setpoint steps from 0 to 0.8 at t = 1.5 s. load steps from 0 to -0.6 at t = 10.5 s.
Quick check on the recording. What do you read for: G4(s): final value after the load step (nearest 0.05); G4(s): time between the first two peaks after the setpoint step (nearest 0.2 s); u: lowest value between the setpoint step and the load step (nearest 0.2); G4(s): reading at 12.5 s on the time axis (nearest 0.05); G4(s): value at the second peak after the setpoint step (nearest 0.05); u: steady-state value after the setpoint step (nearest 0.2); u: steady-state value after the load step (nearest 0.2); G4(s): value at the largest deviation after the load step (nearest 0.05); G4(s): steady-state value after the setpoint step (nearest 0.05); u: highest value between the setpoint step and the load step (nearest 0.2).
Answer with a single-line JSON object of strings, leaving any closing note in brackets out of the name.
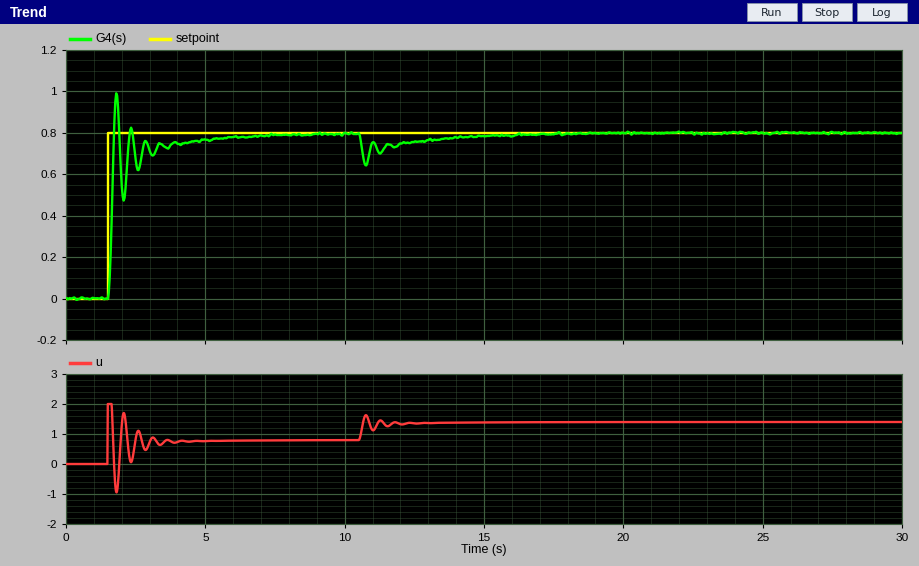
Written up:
{"G4(s): final value after the load step": "0.80", "G4(s): time between the first two peaks after the setpoint step": "0.6 s", "u: lowest value between the setpoint step and the load step": "-1.0", "G4(s): reading at 12.5 s on the time axis": "0.75", "G4(s): value at the second peak after the setpoint step": "0.80", "u: steady-state value after the setpoint step": "0.8", "u: steady-state value after the load step": "1.4", "G4(s): value at the largest deviation after the load step": "0.65", "G4(s): steady-state value after the setpoint step": "0.80", "u: highest value between the setpoint step and the load step": "2.0"}
